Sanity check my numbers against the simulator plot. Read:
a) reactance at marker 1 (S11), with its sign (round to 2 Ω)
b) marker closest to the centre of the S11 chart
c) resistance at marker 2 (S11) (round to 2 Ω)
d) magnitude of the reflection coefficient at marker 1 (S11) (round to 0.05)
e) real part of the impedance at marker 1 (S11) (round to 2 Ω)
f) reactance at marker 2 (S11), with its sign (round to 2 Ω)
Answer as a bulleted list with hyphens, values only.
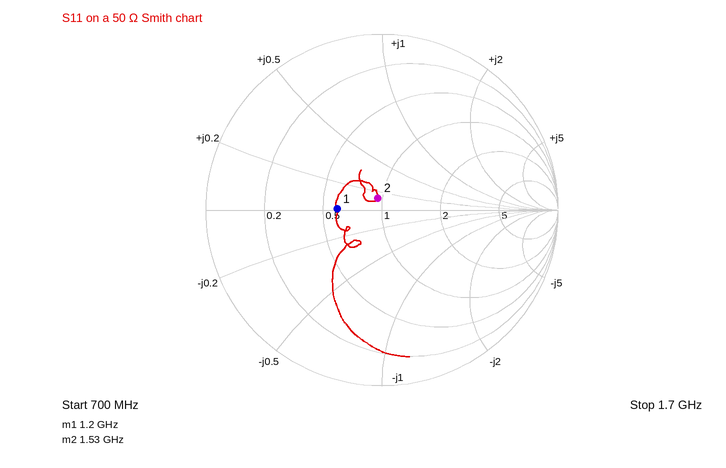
- 0 Ω
- marker 2
- 48 Ω
- 0.25
- 30 Ω
- +6 Ω
